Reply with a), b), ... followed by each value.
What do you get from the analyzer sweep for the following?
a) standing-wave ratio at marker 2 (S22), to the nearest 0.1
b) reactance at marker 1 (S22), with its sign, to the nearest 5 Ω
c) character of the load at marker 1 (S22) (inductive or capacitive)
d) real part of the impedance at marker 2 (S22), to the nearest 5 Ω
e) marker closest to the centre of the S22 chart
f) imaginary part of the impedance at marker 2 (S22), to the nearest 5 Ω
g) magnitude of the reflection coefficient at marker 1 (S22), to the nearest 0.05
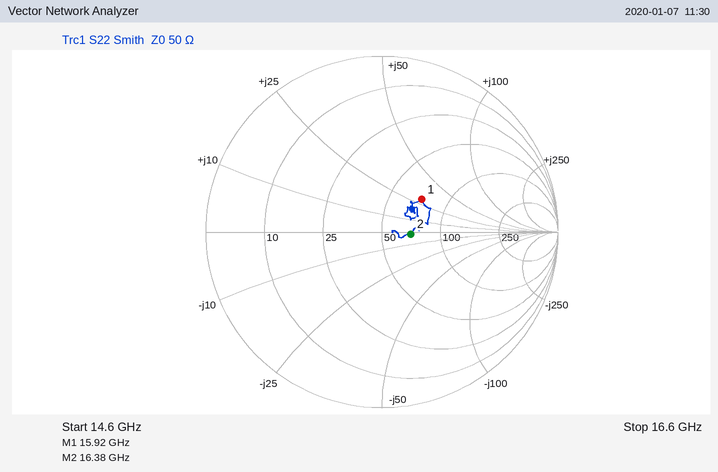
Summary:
a) 1.4
b) +30 Ω
c) inductive
d) 70 Ω
e) marker 2
f) 0 Ω
g) 0.30
